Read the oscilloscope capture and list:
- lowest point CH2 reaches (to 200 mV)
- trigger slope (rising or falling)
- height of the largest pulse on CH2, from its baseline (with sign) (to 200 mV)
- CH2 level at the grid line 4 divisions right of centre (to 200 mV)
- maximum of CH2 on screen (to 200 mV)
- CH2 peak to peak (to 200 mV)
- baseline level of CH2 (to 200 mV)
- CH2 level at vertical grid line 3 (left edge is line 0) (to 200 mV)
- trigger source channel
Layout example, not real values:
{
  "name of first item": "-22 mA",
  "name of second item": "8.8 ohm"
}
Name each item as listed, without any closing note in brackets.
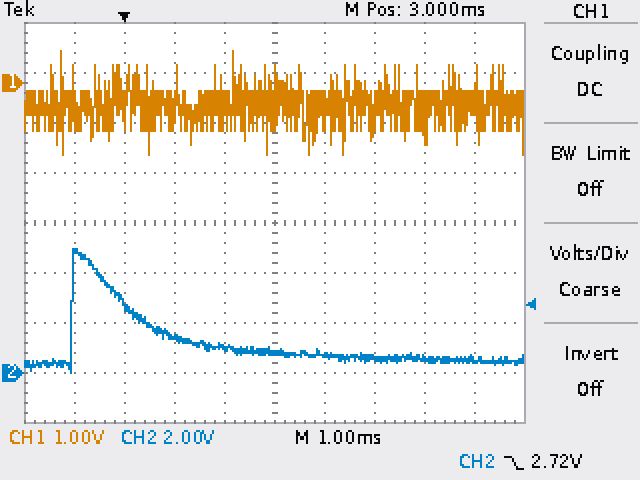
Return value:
{
  "lowest point CH2 reaches": "0.0 V",
  "trigger slope": "falling",
  "height of the largest pulse on CH2, from its baseline (with sign)": "+4.4 V",
  "CH2 level at the grid line 4 divisions right of centre": "600 mV",
  "maximum of CH2 on screen": "5.0 V",
  "CH2 peak to peak": "5.0 V",
  "baseline level of CH2": "600 mV",
  "CH2 level at vertical grid line 3 (left edge is line 0)": "1.4 V",
  "trigger source channel": "CH2"
}
